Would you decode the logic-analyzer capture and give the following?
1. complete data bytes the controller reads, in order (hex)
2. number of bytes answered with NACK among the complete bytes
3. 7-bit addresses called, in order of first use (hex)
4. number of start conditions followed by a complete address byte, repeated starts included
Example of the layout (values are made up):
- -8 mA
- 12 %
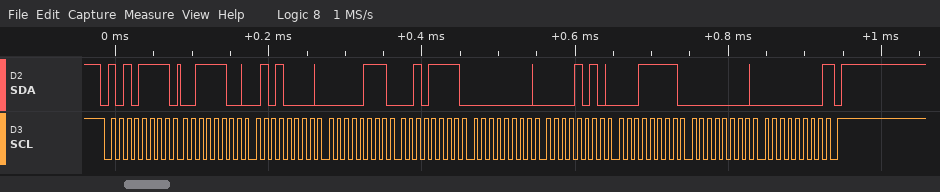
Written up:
- 3C 50 07 2F 00 0A 1F 00 00
- 1
- 0x57
- 1
